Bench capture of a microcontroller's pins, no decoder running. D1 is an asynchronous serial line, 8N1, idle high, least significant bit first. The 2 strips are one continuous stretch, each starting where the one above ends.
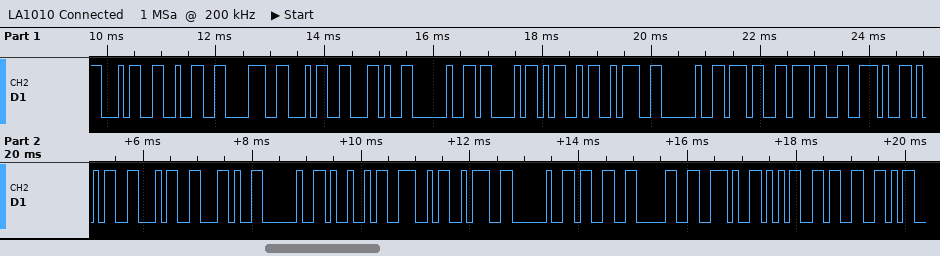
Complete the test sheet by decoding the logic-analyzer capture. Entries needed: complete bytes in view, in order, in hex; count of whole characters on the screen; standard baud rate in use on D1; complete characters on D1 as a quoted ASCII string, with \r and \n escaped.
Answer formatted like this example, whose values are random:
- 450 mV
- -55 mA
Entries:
- 34 32 38 34 2C 20 43 4D 3A 20 37 37 2E 35 34 2C 20 49 4E 3A 20 33 30 2E 35 33
- 26
- 9600 baud
- "4284, CM: 77.54, IN: 30.53"
